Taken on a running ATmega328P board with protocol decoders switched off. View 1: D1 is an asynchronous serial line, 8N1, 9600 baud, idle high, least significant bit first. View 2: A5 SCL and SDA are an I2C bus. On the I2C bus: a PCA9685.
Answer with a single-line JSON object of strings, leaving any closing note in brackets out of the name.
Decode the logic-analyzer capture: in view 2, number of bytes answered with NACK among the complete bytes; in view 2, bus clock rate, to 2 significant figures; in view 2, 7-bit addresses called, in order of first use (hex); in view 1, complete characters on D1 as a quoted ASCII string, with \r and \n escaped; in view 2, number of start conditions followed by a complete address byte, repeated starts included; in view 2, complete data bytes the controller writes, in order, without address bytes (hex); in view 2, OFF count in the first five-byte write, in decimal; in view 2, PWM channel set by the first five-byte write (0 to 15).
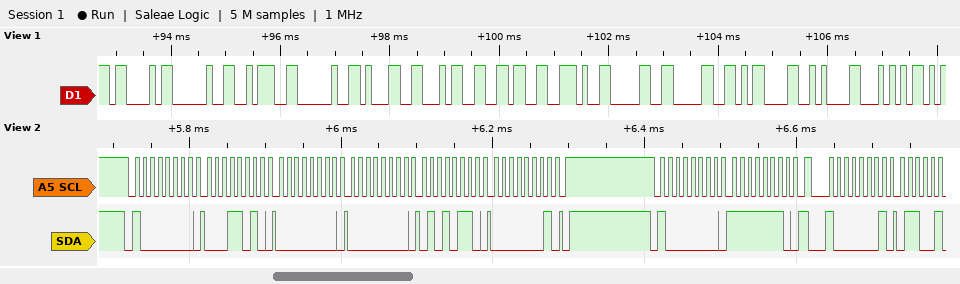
{"in view 2, number of bytes answered with NACK among the complete bytes": "0", "in view 2, bus clock rate, to 2 significant figures": "100 kHz", "in view 2, 7-bit addresses called, in order of first use": "0x40", "in view 1, complete characters on D1 as a quoted ASCII string, with \\r and \\n escaped": "\"C : 146.00\\r\\nT\"", "in view 2, number of start conditions followed by a complete address byte, repeated starts included": "3", "in view 2, complete data bytes the controller writes, in order, without address bytes": "1A 00 00 56 01 FE", "in view 2, OFF count in the first five-byte write, in decimal": "342", "in view 2, PWM channel set by the first five-byte write": "5"}
